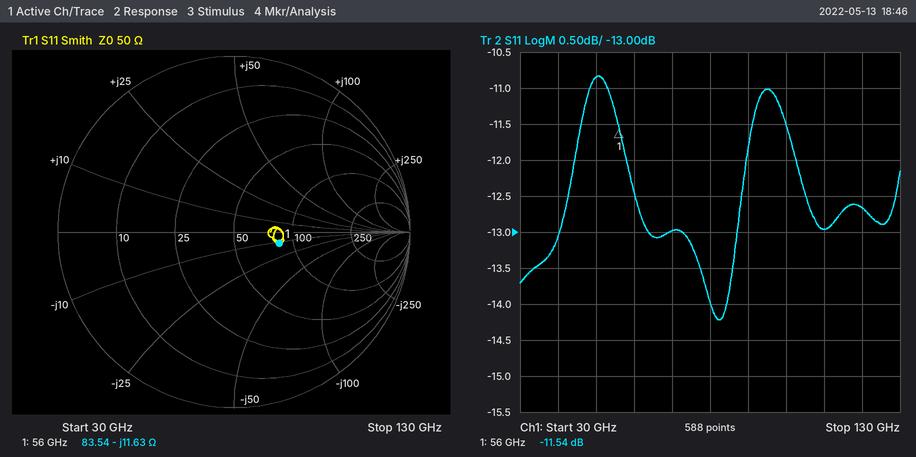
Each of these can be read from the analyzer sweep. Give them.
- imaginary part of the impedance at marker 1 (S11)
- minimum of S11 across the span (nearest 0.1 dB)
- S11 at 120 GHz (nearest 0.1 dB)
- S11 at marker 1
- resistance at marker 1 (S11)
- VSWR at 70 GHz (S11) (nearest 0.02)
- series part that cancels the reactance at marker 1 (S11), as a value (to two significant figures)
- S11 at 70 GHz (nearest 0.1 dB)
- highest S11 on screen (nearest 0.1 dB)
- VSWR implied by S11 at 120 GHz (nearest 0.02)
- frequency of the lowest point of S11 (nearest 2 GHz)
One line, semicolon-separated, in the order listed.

-11.63 Ω; -14.2 dB; -12.7 dB; -11.54 dB; 83.54 Ω; 1.58; 33 pH; -13.0 dB; -10.8 dB; 1.60; 82 GHz
